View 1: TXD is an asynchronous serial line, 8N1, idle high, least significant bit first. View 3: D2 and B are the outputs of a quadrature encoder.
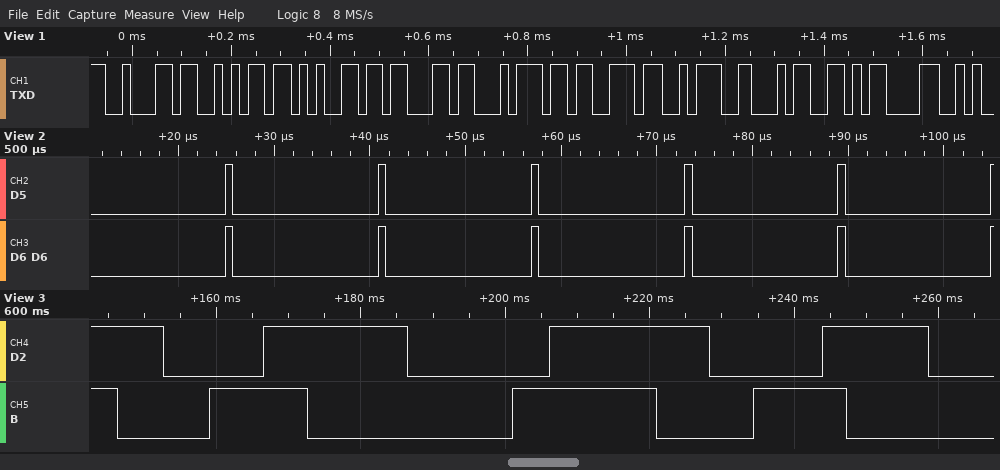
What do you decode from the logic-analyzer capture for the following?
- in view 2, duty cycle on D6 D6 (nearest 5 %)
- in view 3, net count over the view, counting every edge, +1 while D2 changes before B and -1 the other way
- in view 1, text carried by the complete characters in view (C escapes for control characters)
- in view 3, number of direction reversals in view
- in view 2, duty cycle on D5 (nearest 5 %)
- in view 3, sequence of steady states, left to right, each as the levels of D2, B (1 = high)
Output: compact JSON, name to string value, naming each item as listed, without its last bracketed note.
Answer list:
{"in view 2, duty cycle on D6 D6": "5 %", "in view 3, net count over the view, counting every edge, +1 while D2 changes before B and -1 the other way": "-14", "in view 1, text carried by the complete characters in view": "\"bjects:4\\r\"", "in view 3, number of direction reversals in view": "0", "in view 2, duty cycle on D5": "5 %", "in view 3, sequence of steady states, left to right, each as the levels of D2, B": "11 10 00 01 11 10 00 01 11 10 00 01 11 10 00"}
